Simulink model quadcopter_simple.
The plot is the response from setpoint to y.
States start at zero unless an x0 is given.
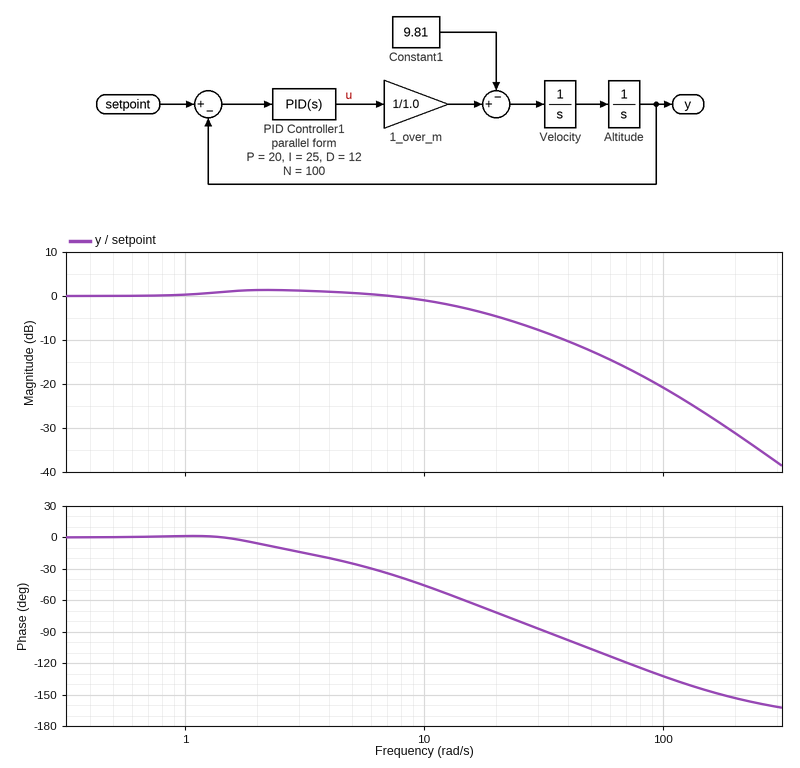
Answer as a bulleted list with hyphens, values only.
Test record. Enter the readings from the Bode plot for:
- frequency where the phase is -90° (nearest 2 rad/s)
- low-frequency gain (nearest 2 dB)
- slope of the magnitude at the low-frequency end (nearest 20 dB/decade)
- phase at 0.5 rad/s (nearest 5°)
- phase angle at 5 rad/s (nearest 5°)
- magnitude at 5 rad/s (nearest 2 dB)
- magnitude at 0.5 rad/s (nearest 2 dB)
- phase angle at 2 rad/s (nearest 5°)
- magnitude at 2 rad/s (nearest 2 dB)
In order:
- 32 rad/s
- 0 dB
- 0 dB/decade
- 0°
- -25°
- 0 dB
- 0 dB
- -5°
- 2 dB
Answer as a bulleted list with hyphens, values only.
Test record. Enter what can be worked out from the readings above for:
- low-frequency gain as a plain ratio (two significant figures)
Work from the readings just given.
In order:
- 1.0
